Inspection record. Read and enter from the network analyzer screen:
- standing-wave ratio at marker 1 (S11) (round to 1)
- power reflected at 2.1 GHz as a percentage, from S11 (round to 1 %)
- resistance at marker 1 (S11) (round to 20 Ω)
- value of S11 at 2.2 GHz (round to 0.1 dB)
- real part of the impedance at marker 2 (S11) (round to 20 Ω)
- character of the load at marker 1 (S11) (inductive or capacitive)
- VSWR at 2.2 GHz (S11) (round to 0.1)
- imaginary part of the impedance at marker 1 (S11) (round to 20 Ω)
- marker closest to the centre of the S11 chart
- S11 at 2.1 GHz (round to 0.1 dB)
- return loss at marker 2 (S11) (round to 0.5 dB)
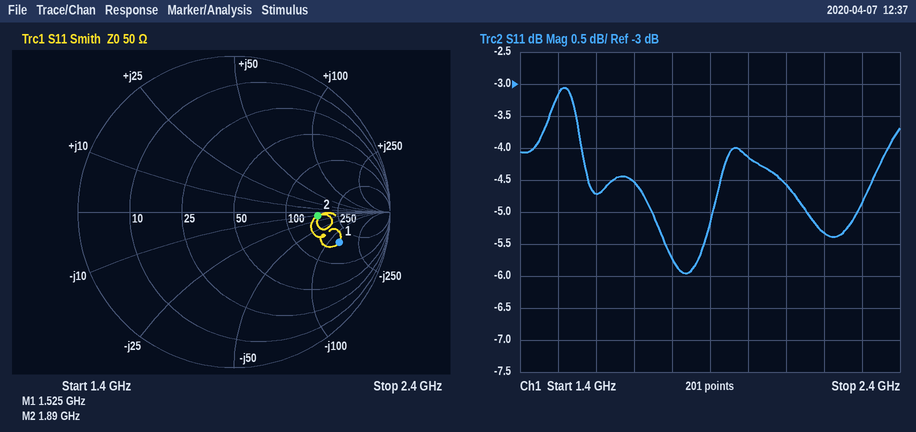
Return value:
6
35 %
180 Ω
-5.3 dB
160 Ω
capacitive
3.4
-140 Ω
marker 2
-4.6 dB
5.5 dB
